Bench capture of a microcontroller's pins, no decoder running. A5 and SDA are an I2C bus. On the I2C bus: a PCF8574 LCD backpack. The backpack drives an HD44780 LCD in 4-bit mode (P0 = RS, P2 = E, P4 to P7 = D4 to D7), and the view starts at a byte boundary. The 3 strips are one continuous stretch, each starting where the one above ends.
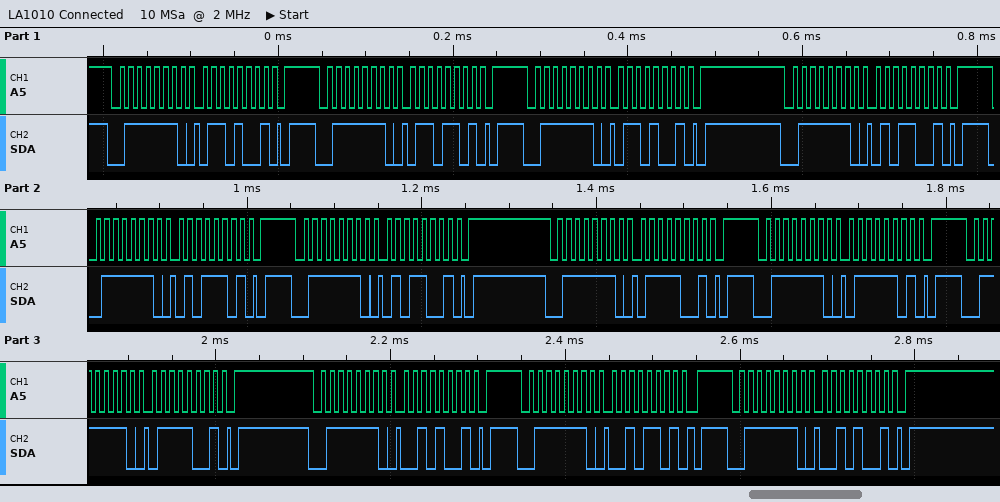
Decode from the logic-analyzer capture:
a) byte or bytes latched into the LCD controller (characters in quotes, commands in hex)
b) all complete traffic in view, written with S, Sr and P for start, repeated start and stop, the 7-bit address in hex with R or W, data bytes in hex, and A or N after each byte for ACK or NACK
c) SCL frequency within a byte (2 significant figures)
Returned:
'e' 'r'
S 3FW A 69 A P S 3FW A 6D A P S 3FW A 69 A P S 3FW A 59 A P S 3FW A 5D A P S 3FW A 59 A P S 3FW A 79 A P S 3FW A 7D A P S 3FW A 79 A P S 3FW A 29 A P S 3FW A 2D A P S 3FW A 29 A P
100 kHz
